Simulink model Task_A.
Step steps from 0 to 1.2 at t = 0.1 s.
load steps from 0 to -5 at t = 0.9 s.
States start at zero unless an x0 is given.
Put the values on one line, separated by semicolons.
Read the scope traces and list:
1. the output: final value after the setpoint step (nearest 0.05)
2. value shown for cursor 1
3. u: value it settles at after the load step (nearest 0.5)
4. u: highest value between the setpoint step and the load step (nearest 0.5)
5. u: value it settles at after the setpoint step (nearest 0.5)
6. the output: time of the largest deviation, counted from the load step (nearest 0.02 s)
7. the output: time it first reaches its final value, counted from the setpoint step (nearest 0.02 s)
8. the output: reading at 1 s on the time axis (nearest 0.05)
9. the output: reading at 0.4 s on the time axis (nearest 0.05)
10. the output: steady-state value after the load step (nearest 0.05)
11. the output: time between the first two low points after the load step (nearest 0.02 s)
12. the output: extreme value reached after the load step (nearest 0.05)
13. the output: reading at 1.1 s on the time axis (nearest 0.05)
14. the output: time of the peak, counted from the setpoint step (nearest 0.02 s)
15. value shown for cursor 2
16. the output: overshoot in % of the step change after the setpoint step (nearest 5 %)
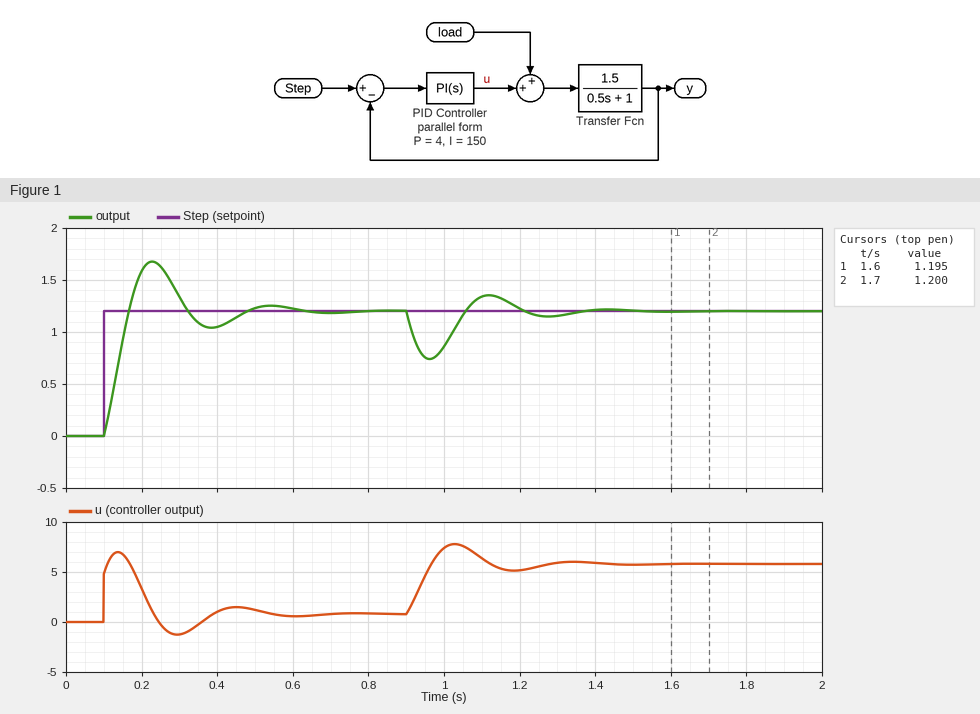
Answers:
1.20; 1.195; 6.0; 7.0; 1.0; 0.06 s; 0.06 s; 0.85; 1.05; 1.20; 0.32 s; 0.75; 1.35; 0.12 s; 1.200; 40 %
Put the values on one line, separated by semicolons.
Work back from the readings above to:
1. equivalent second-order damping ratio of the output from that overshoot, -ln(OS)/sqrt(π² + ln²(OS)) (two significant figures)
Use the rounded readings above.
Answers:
0.28
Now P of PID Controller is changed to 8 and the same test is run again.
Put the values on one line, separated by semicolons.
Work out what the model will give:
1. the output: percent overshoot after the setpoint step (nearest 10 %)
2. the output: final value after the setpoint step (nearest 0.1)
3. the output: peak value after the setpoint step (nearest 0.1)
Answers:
20 %; 1.2; 1.5
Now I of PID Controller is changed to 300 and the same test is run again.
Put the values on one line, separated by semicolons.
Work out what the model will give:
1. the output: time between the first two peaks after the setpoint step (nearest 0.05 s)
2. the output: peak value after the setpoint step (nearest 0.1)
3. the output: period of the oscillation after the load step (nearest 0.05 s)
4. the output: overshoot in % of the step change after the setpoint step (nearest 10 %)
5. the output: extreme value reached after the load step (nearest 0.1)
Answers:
0.20 s; 1.8; 0.20 s; 50 %; 0.8
